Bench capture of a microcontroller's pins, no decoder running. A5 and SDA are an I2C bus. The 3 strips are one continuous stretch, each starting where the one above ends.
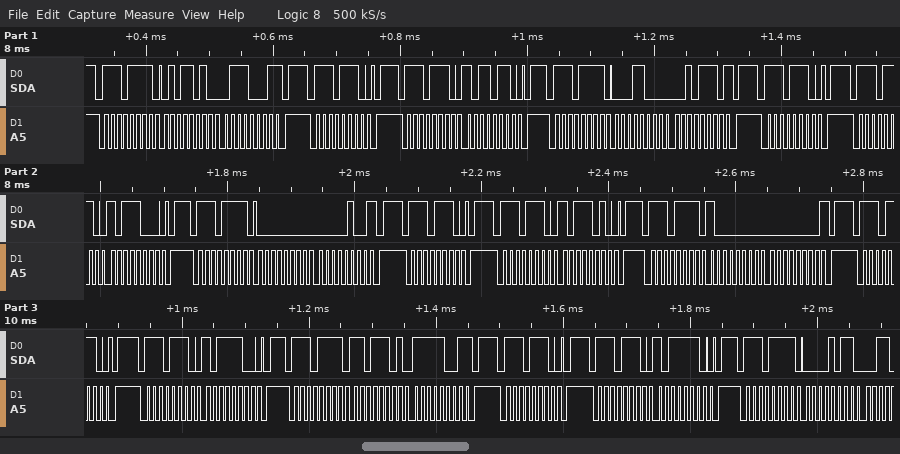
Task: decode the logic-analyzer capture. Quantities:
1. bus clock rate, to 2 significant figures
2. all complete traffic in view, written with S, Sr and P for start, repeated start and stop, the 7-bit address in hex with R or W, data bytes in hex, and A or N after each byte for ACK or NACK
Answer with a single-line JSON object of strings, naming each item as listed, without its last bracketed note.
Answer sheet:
{"bus clock rate, to 2 significant figures": "100 kHz", "all complete traffic in view, written with S, Sr and P for start, repeated start and stop, the 7-bit address in hex with R or W, data bytes in hex, and A or N after each byte for ACK or NACK": "S 77R A 5A A 71 N P S 77W A P S 77W A B6 A P S 77R A 18 A 2E N P S 77W A P S 77W A B8 A P S 77R A 00 A 04 N P S 77W A P S 77W A BA A P S 77R A 80 A 00 N P S 77W A P S 77W A BC A P S 77R A DD A F9 N P S 77W A P S 77W A BE A P S 77R A 0B A"}
